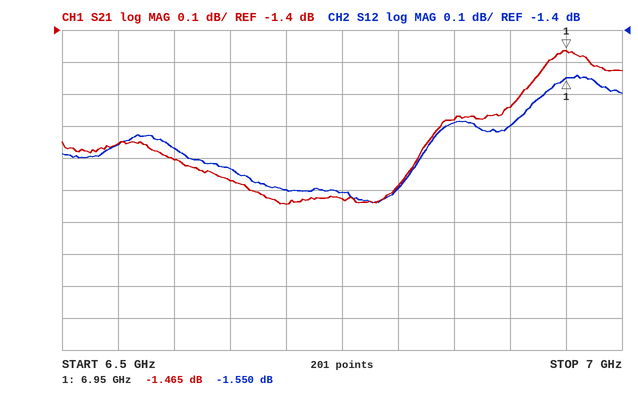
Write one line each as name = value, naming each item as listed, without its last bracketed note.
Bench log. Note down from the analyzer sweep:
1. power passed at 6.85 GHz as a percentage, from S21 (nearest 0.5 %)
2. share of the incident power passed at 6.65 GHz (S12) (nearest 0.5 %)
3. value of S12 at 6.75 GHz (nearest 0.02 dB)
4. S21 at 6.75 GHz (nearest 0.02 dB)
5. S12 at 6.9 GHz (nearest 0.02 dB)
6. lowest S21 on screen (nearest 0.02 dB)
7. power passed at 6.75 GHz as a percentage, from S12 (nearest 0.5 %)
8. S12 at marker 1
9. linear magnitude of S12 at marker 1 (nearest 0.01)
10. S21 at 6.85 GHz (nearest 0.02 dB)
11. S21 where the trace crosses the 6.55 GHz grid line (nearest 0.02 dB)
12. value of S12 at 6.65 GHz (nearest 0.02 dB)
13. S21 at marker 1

power passed at 6.85 GHz as a percentage, from S21 = 68.0 %
share of the incident power passed at 6.65 GHz (S12) = 65.5 %
value of S12 at 6.75 GHz = -1.90 dB
S21 at 6.75 GHz = -1.92 dB
S12 at 6.9 GHz = -1.70 dB
lowest S21 on screen = -1.94 dB
power passed at 6.75 GHz as a percentage, from S12 = 64.5 %
S12 at marker 1 = -1.550 dB
linear magnitude of S12 at marker 1 = 0.84
S21 at 6.85 GHz = -1.68 dB
S21 where the trace crosses the 6.55 GHz grid line = -1.76 dB
value of S12 at 6.65 GHz = -1.84 dB
S21 at marker 1 = -1.465 dB
